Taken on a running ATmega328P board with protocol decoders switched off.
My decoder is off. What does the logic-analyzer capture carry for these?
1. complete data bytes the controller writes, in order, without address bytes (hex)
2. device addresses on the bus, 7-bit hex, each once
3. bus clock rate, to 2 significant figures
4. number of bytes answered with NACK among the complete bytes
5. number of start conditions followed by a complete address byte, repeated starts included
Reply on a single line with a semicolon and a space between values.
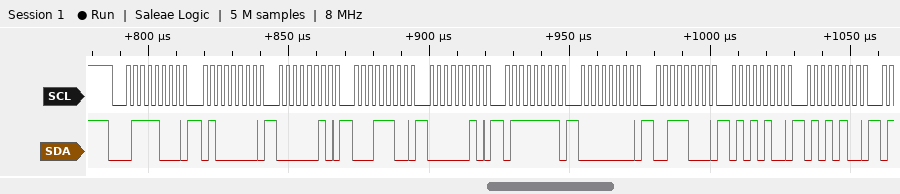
40 02 1C 02 7F 00 38 54 54; 0x3C; 400 kHz; 0; 1
